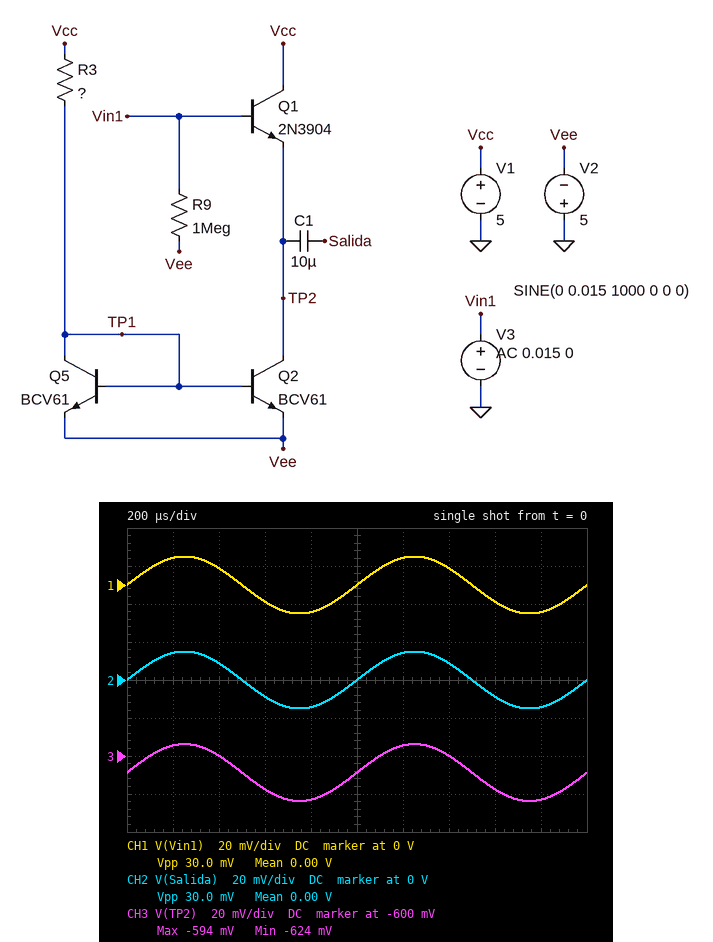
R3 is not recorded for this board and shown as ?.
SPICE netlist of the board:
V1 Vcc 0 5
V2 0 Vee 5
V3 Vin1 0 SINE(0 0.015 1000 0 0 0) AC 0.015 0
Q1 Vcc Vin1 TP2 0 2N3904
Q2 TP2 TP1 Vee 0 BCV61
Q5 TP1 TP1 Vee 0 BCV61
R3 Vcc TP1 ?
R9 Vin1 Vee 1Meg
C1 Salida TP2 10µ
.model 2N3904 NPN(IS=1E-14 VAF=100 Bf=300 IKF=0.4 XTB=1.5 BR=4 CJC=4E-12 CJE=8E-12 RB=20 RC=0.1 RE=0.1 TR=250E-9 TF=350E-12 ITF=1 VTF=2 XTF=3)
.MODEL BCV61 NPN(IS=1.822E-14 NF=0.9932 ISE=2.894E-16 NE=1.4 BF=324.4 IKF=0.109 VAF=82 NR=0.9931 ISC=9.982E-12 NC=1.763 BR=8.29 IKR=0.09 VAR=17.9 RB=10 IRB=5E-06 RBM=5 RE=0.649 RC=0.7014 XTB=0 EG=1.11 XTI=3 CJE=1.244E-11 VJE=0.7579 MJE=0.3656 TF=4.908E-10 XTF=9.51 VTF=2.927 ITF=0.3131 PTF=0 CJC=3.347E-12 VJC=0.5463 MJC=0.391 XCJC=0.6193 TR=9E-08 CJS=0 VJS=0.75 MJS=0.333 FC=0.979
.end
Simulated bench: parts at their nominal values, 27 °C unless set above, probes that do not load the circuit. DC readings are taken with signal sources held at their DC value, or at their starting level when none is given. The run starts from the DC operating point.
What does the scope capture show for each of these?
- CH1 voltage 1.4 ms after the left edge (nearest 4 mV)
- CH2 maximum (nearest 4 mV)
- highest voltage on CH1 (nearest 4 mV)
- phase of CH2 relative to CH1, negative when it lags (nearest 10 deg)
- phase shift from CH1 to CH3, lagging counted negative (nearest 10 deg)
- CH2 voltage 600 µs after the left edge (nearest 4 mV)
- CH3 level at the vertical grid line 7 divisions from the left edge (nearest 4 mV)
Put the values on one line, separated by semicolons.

8 mV; 16 mV; 16 mV; 0 deg; 0 deg; -8 mV; -600 mV
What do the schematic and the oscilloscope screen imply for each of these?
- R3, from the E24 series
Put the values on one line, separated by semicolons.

56 kΩ
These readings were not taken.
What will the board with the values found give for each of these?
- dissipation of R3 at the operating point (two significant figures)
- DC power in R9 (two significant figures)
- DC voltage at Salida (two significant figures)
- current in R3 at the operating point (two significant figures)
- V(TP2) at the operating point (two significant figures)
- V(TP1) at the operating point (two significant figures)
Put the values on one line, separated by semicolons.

1.6 mW; 25 µW; -610 mV; 170 µA; -610 mV; -4.4 V
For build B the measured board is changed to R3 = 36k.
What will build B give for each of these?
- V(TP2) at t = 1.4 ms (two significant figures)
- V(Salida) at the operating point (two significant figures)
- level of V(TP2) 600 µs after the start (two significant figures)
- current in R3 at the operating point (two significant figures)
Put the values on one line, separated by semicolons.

-610 mV; -620 mV; -630 mV; 260 µA
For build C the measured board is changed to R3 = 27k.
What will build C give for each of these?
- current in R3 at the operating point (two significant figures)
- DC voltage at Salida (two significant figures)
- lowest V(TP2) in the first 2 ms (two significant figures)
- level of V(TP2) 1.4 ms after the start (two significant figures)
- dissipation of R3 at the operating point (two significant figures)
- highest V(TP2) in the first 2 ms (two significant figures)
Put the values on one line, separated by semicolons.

350 µA; -630 mV; -640 mV; -620 mV; 3.3 mW; -610 mV
